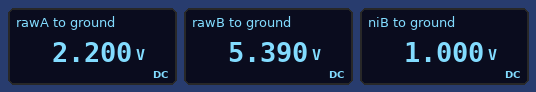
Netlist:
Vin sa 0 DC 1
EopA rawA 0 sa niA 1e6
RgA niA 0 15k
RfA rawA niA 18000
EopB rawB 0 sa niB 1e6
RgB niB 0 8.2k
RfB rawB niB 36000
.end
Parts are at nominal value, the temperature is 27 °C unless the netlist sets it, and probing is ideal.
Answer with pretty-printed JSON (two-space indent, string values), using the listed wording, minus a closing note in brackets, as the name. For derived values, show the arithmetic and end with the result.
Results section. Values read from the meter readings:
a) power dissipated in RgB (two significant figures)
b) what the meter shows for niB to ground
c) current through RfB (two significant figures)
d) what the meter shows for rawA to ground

{
  "power dissipated in RgB": "(1 V)^2 / 8.2 kΩ = 120 µW",
  "what the meter shows for niB to ground": "1.000 V",
  "current through RfB": "(5.39 V - 1 V) / 36 kΩ = 120 µA",
  "what the meter shows for rawA to ground": "2.200 V"
}
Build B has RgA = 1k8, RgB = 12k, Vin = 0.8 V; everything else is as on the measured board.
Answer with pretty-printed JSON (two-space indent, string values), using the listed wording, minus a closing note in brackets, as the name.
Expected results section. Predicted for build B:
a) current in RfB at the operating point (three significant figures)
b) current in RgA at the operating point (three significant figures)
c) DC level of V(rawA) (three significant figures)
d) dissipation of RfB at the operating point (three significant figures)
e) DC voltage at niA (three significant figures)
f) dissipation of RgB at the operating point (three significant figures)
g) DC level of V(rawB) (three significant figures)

{
  "current in RfB at the operating point": "66.7 µA",
  "current in RgA at the operating point": "444 µA",
  "DC level of V(rawA)": "8.80 V",
  "dissipation of RfB at the operating point": "160 µW",
  "DC voltage at niA": "800 mV",
  "dissipation of RgB at the operating point": "53.3 µW",
  "DC level of V(rawB)": "3.20 V"
}
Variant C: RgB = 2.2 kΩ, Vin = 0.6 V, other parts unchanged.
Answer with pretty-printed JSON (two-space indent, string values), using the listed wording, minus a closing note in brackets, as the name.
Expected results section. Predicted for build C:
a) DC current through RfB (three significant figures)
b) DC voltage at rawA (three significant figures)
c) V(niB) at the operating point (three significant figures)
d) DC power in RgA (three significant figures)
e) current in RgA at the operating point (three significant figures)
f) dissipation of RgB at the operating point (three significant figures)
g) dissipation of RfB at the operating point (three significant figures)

{
  "DC current through RfB": "273 µA",
  "DC voltage at rawA": "1.32 V",
  "V(niB) at the operating point": "600 mV",
  "DC power in RgA": "24.0 µW",
  "current in RgA at the operating point": "40.0 µA",
  "dissipation of RgB at the operating point": "164 µW",
  "dissipation of RfB at the operating point": "2.68 mW"
}
